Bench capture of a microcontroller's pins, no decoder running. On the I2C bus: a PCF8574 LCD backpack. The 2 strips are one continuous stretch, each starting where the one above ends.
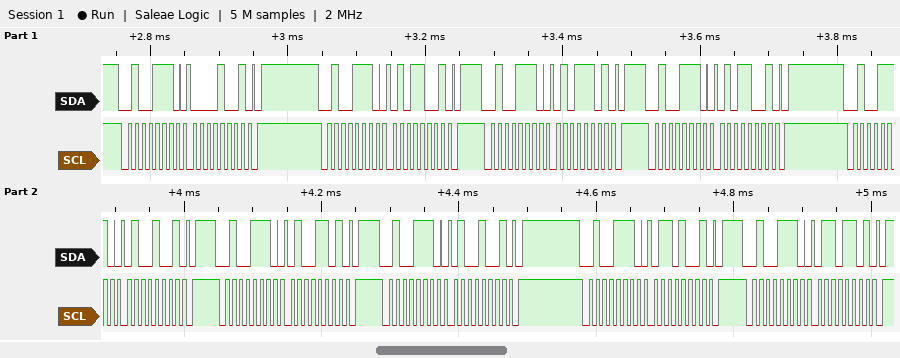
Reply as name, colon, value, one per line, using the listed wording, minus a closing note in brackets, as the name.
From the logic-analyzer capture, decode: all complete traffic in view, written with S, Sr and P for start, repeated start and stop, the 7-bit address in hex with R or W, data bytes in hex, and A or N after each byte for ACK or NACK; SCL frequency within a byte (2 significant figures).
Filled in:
all complete traffic in view, written with S, Sr and P for start, repeated start and stop, the 7-bit address in hex with R or W, data bytes in hex, and A or N after each byte for ACK or NACK: S 27W A 09 A P S 27W A 59 A P S 27W A 5D A P S 27W A 59 A P S 27W A 49 A P S 27W A 4D A P S 27W A 49 A P S 27W A 69 A P S 27W A 6D A P
SCL frequency within a byte: 100 kHz
